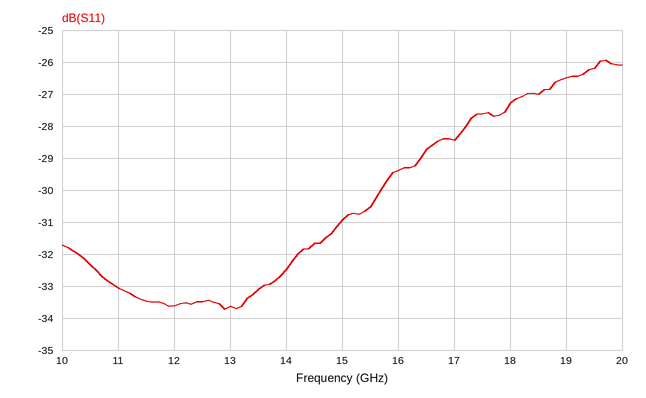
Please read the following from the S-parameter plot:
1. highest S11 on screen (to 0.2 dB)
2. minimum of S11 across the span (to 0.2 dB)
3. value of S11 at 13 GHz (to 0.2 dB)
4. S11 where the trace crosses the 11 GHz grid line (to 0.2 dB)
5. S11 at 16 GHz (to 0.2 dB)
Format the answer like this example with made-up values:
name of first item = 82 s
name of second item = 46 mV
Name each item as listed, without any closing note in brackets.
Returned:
highest S11 on screen = -26.0 dB
minimum of S11 across the span = -33.8 dB
value of S11 at 13 GHz = -33.6 dB
S11 where the trace crosses the 11 GHz grid line = -33.0 dB
S11 at 16 GHz = -29.4 dB
